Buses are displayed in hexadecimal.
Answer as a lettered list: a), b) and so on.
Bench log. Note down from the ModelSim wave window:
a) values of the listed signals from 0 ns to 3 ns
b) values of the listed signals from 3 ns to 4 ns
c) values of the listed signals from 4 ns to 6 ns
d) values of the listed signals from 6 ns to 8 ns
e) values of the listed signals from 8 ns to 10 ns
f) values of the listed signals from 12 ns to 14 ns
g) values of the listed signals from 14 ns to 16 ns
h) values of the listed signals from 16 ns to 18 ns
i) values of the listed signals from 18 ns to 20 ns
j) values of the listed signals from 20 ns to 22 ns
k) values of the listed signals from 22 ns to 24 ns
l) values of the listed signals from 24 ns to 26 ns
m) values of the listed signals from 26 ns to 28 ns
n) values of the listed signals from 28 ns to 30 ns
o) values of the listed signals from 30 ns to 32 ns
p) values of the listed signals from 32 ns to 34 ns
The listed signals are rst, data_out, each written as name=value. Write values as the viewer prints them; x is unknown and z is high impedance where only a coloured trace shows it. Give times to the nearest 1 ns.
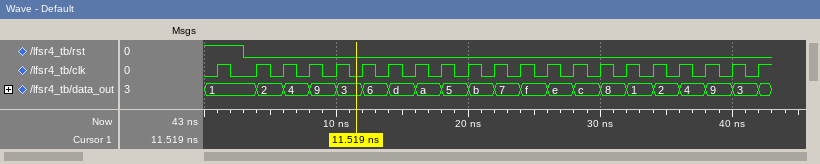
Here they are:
a) rst=1, data_out=1
b) rst=0, data_out=1
c) rst=0, data_out=2
d) rst=0, data_out=4
e) rst=0, data_out=9
f) rst=0, data_out=6
g) rst=0, data_out=d
h) rst=0, data_out=a
i) rst=0, data_out=5
j) rst=0, data_out=b
k) rst=0, data_out=7
l) rst=0, data_out=f
m) rst=0, data_out=e
n) rst=0, data_out=c
o) rst=0, data_out=8
p) rst=0, data_out=1
